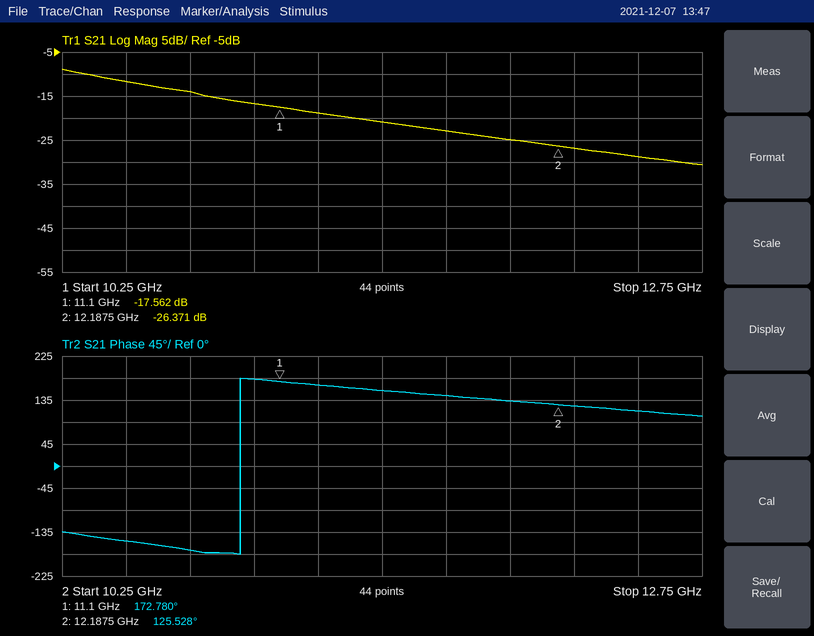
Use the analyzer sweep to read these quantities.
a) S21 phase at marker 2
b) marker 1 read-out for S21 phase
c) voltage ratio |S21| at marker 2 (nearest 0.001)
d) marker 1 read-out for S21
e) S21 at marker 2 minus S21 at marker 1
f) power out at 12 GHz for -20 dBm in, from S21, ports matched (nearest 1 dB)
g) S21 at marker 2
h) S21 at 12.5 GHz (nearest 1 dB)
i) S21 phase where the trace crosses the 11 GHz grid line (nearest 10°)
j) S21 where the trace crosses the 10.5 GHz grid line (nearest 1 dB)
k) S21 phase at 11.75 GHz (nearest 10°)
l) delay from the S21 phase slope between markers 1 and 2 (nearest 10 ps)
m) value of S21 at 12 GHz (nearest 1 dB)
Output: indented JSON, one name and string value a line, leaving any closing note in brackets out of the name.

{
  "S21 phase at marker 2": "125.528°",
  "marker 1 read-out for S21 phase": "172.780°",
  "voltage ratio |S21| at marker 2": "0.048",
  "marker 1 read-out for S21": "-17.562 dB",
  "S21 at marker 2 minus S21 at marker 1": "-8.809 dB",
  "power out at 12 GHz for -20 dBm in, from S21, ports matched": "-45 dBm",
  "S21 at marker 2": "-26.371 dB",
  "S21 at 12.5 GHz": "-29 dB",
  "S21 phase where the trace crosses the 11 GHz grid line": "180°",
  "S21 where the trace crosses the 10.5 GHz grid line": "-12 dB",
  "S21 phase at 11.75 GHz": "140°",
  "delay from the S21 phase slope between markers 1 and 2": "120 ps",
  "value of S21 at 12 GHz": "-25 dB"
}
